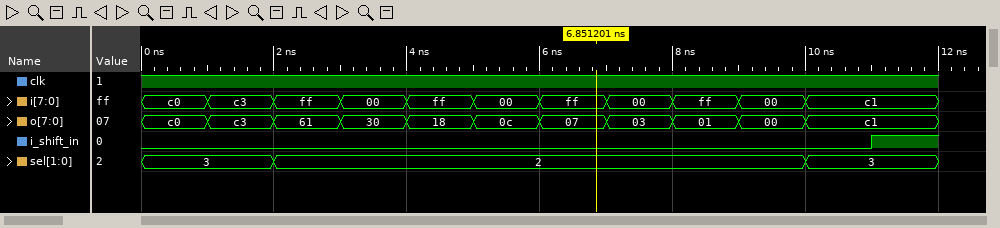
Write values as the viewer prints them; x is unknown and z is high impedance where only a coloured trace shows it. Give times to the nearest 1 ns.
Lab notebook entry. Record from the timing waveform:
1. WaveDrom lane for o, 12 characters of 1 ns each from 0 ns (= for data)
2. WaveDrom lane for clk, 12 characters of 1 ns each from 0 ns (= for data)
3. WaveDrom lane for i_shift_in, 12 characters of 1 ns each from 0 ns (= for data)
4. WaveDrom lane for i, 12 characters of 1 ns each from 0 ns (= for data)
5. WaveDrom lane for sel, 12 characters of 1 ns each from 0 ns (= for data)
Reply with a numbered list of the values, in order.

1. {name: 'o', wave: '===========.', data: 'c0 c3 61 30 18 0c 07 03 01 00 c1'}
2. {name: 'clk', wave: '1...........'}
3. {name: 'i_shift_in', wave: '0..........1'}
4. {name: 'i', wave: '===========.', data: 'c0 c3 ff 00 ff 00 ff 00 ff 00 c1'}
5. {name: 'sel', wave: '=.=.......=.', data: '3 2 3'}
